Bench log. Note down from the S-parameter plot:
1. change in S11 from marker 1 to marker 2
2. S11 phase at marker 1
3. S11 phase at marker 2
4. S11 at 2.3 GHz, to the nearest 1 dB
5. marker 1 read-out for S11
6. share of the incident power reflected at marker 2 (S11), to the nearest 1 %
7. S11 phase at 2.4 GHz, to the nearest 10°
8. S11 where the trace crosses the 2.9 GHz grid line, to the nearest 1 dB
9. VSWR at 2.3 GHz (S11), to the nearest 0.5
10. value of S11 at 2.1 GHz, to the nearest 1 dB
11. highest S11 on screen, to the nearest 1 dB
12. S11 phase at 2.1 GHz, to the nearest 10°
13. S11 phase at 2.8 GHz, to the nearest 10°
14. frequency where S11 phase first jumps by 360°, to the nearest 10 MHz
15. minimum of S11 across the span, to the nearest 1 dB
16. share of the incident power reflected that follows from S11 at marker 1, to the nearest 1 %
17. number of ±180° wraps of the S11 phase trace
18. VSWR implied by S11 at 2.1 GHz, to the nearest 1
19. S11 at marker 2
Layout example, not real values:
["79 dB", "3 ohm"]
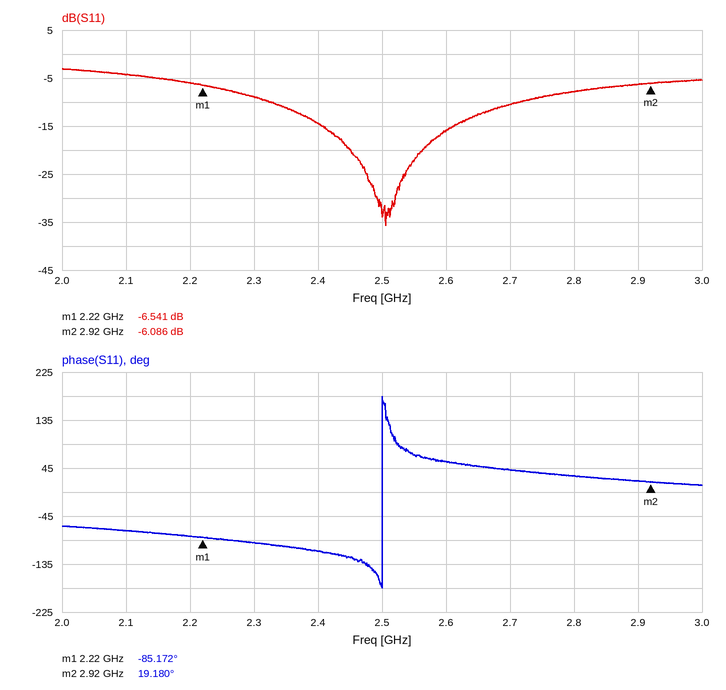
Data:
["0.455 dB", "-85.172°", "19.180°", "-9 dB", "-6.541 dB", "25 %", "-110°", "-6 dB", "2.0", "-4 dB", "-3 dB", "-70°", "30°", "2.50 GHz", "-36 dB", "22 %", "1", "4", "-6.086 dB"]
